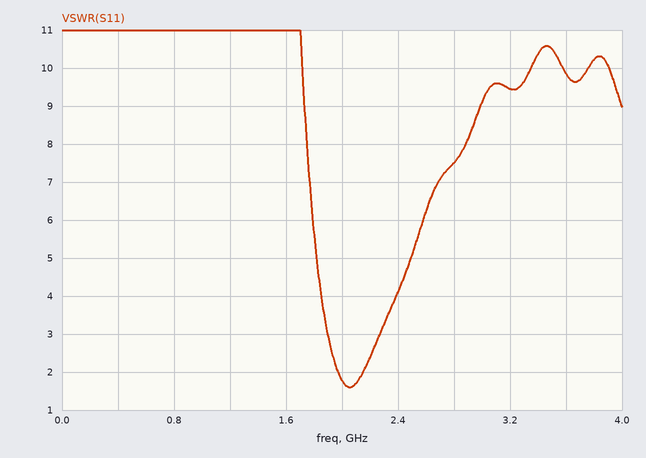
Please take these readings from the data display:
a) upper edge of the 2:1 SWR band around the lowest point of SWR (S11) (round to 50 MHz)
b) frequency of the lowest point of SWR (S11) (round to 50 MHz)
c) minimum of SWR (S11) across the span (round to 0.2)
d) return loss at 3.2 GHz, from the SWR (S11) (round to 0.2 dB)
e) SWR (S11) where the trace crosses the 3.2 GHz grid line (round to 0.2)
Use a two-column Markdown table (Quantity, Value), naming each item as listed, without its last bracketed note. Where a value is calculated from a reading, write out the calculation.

| Quantity | Value |
|---|---|
| upper edge of the 2:1 SWR band around the lowest point of SWR (S11) | 2.15 GHz |
| frequency of the lowest point of SWR (S11) | 2.05 GHz |
| minimum of SWR (S11) across the span | 1.6 |
| return loss at 3.2 GHz, from the SWR (S11) | −20 log10((9.4 − 1)/(9.4 + 1)) ≈ 1.86 dB, so 1.8 dB to the nearest 0.2 dB |
| SWR (S11) where the trace crosses the 3.2 GHz grid line | 9.4 |
